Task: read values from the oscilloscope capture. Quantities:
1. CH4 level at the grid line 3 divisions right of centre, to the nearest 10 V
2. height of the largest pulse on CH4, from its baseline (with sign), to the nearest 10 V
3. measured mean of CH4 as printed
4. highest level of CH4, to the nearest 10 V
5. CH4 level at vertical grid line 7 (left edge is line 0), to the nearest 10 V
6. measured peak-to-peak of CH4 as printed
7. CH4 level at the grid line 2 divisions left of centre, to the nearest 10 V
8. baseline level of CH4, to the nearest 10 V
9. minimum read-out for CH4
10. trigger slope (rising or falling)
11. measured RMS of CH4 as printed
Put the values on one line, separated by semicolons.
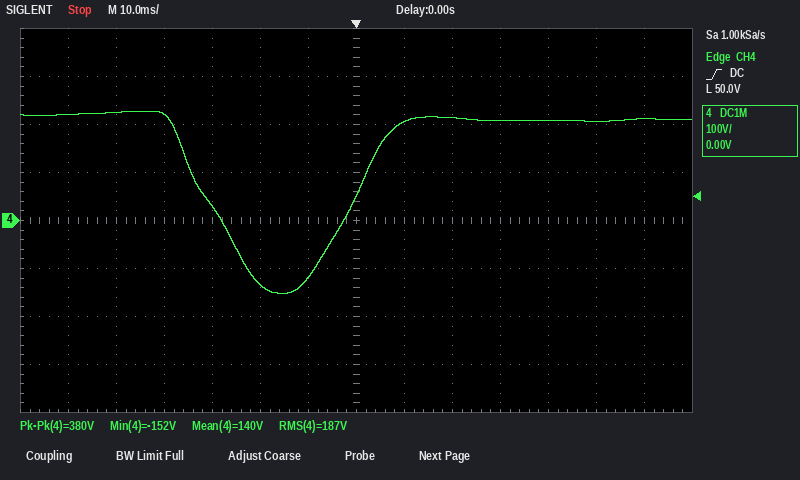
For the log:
210 V; -360 V; 140 V; 230 V; 50 V; 380 V; -130 V; 210 V; -152 V; rising; 187 V
